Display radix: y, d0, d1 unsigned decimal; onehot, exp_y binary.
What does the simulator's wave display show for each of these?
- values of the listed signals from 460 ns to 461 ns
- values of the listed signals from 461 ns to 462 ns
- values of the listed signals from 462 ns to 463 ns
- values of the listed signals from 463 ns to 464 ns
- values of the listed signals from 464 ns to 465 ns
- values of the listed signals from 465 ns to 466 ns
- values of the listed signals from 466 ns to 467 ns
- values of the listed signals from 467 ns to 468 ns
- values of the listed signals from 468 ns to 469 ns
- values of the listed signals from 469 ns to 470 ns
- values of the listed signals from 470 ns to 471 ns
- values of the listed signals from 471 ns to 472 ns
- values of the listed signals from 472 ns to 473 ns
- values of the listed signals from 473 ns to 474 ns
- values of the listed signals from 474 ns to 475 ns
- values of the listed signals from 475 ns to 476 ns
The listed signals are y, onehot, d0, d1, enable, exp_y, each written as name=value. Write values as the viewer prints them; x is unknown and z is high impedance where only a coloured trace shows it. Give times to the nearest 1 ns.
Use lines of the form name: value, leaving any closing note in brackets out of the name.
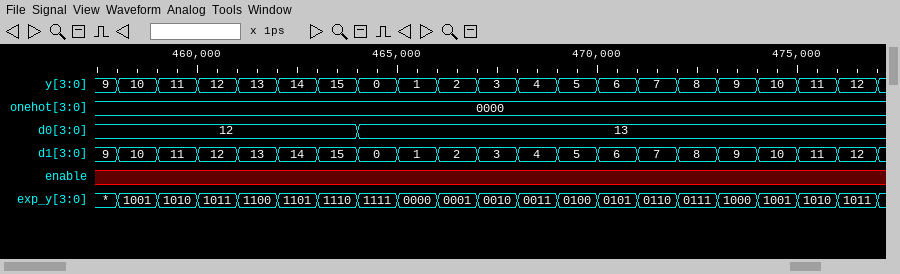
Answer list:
values of the listed signals from 460 ns to 461 ns: y=12, onehot=0000, d0=12, d1=12, enable=x, exp_y=1011
values of the listed signals from 461 ns to 462 ns: y=13, onehot=0000, d0=12, d1=13, enable=x, exp_y=1100
values of the listed signals from 462 ns to 463 ns: y=14, onehot=0000, d0=12, d1=14, enable=x, exp_y=1101
values of the listed signals from 463 ns to 464 ns: y=15, onehot=0000, d0=12, d1=15, enable=x, exp_y=1110
values of the listed signals from 464 ns to 465 ns: y=0, onehot=0000, d0=13, d1=0, enable=x, exp_y=1111
values of the listed signals from 465 ns to 466 ns: y=1, onehot=0000, d0=13, d1=1, enable=x, exp_y=0000
values of the listed signals from 466 ns to 467 ns: y=2, onehot=0000, d0=13, d1=2, enable=x, exp_y=0001
values of the listed signals from 467 ns to 468 ns: y=3, onehot=0000, d0=13, d1=3, enable=x, exp_y=0010
values of the listed signals from 468 ns to 469 ns: y=4, onehot=0000, d0=13, d1=4, enable=x, exp_y=0011
values of the listed signals from 469 ns to 470 ns: y=5, onehot=0000, d0=13, d1=5, enable=x, exp_y=0100
values of the listed signals from 470 ns to 471 ns: y=6, onehot=0000, d0=13, d1=6, enable=x, exp_y=0101
values of the listed signals from 471 ns to 472 ns: y=7, onehot=0000, d0=13, d1=7, enable=x, exp_y=0110
values of the listed signals from 472 ns to 473 ns: y=8, onehot=0000, d0=13, d1=8, enable=x, exp_y=0111
values of the listed signals from 473 ns to 474 ns: y=9, onehot=0000, d0=13, d1=9, enable=x, exp_y=1000
values of the listed signals from 474 ns to 475 ns: y=10, onehot=0000, d0=13, d1=10, enable=x, exp_y=1001
values of the listed signals from 475 ns to 476 ns: y=11, onehot=0000, d0=13, d1=11, enable=x, exp_y=1010
